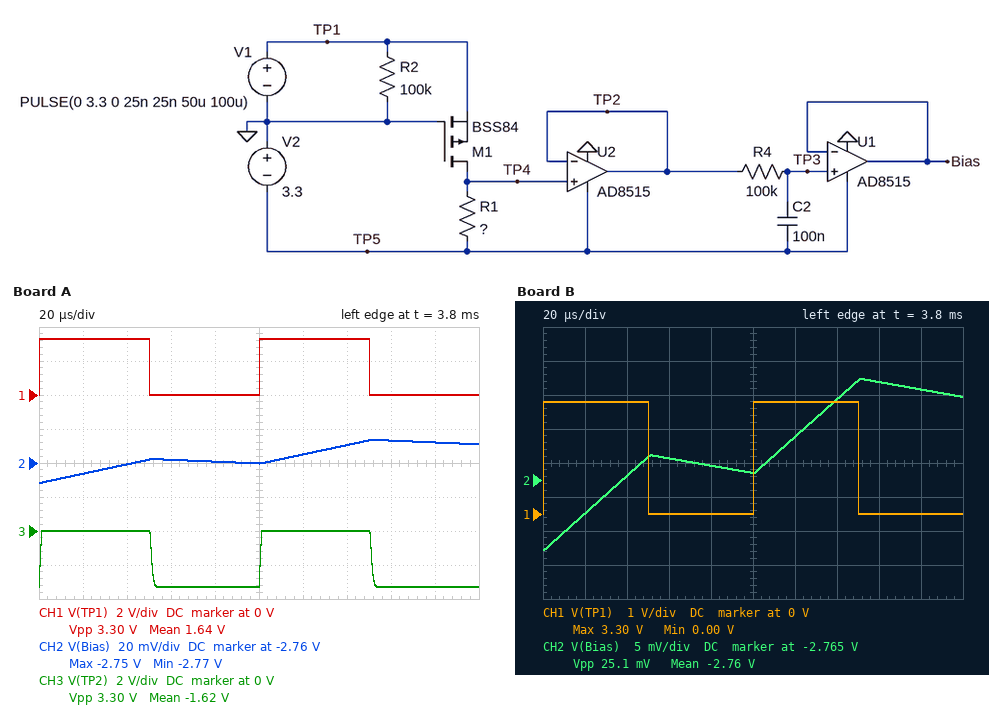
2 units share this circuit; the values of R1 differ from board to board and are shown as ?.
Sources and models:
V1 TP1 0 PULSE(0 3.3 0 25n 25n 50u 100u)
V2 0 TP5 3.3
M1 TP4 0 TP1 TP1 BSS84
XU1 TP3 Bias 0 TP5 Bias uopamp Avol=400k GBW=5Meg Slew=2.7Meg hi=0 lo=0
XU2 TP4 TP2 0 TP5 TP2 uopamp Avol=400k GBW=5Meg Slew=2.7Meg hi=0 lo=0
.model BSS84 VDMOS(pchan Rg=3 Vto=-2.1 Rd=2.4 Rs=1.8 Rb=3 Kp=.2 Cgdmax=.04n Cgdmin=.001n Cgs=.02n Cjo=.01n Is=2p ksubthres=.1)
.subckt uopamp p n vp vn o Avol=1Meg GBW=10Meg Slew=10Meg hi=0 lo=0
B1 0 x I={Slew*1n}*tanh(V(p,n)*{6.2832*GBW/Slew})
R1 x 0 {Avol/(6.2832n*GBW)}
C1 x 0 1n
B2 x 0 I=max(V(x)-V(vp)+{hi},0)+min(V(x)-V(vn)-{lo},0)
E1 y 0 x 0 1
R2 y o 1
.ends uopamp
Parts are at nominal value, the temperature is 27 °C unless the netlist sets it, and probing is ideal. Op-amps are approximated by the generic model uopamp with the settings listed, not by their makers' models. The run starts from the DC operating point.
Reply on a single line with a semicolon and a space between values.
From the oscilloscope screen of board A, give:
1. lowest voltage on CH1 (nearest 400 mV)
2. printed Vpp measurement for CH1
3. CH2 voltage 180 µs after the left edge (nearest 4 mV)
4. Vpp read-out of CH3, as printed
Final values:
0 V; 3.30 V; -2.748 V; 3.30 V
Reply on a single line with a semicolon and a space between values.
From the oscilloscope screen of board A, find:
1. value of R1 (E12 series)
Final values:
56 kΩ
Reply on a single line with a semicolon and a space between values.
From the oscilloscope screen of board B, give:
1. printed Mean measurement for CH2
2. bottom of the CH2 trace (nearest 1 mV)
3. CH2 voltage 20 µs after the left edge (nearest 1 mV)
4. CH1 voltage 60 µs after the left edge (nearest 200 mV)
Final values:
-2.76 V; -2.775 V; -2.770 V; 0 V
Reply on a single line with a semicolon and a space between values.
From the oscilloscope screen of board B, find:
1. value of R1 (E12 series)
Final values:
39 kΩ
